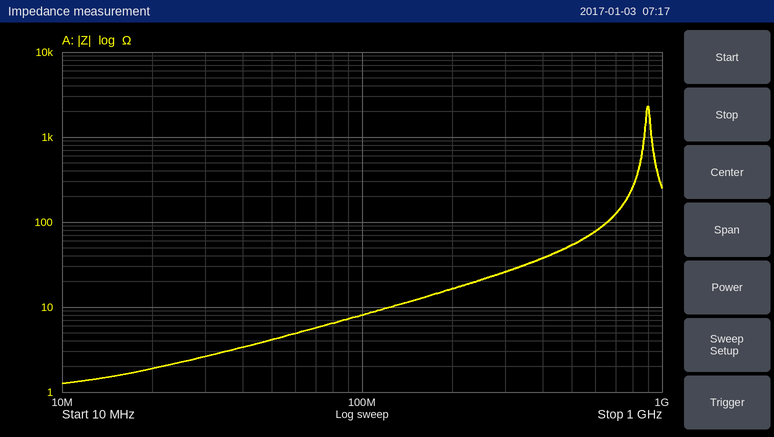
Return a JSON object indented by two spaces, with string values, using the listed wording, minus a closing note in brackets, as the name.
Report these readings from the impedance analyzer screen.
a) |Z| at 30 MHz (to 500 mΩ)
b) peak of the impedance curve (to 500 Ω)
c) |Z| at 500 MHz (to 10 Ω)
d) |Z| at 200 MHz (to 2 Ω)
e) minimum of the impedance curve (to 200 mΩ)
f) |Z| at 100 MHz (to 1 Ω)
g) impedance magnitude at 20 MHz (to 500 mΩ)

{
  "|Z| at 30 MHz": "2.5 Ω",
  "peak of the impedance curve": "2.5 kΩ",
  "|Z| at 500 MHz": "50 Ω",
  "|Z| at 200 MHz": "16 Ω",
  "minimum of the impedance curve": "1.2 Ω",
  "|Z| at 100 MHz": "8 Ω",
  "impedance magnitude at 20 MHz": "2.0 Ω"
}
